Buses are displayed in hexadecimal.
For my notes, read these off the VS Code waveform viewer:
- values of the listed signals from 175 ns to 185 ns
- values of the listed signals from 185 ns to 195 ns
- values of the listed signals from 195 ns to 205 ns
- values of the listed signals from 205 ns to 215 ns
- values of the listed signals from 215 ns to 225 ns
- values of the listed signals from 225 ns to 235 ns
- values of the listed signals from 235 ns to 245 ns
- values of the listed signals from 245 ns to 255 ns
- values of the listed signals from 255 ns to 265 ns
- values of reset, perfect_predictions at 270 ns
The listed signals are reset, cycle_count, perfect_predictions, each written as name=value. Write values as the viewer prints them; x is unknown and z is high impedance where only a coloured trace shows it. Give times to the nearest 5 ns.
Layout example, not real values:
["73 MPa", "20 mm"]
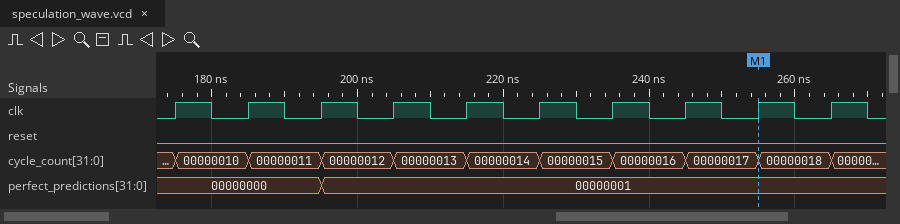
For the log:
["reset=0, cycle_count=00000010, perfect_predictions=00000000", "reset=0, cycle_count=00000011, perfect_predictions=00000000", "reset=0, cycle_count=00000012, perfect_predictions=00000001", "reset=0, cycle_count=00000013, perfect_predictions=00000001", "reset=0, cycle_count=00000014, perfect_predictions=00000001", "reset=0, cycle_count=00000015, perfect_predictions=00000001", "reset=0, cycle_count=00000016, perfect_predictions=00000001", "reset=0, cycle_count=00000017, perfect_predictions=00000001", "reset=0, cycle_count=00000018, perfect_predictions=00000001", "reset=0, perfect_predictions=00000001"]
